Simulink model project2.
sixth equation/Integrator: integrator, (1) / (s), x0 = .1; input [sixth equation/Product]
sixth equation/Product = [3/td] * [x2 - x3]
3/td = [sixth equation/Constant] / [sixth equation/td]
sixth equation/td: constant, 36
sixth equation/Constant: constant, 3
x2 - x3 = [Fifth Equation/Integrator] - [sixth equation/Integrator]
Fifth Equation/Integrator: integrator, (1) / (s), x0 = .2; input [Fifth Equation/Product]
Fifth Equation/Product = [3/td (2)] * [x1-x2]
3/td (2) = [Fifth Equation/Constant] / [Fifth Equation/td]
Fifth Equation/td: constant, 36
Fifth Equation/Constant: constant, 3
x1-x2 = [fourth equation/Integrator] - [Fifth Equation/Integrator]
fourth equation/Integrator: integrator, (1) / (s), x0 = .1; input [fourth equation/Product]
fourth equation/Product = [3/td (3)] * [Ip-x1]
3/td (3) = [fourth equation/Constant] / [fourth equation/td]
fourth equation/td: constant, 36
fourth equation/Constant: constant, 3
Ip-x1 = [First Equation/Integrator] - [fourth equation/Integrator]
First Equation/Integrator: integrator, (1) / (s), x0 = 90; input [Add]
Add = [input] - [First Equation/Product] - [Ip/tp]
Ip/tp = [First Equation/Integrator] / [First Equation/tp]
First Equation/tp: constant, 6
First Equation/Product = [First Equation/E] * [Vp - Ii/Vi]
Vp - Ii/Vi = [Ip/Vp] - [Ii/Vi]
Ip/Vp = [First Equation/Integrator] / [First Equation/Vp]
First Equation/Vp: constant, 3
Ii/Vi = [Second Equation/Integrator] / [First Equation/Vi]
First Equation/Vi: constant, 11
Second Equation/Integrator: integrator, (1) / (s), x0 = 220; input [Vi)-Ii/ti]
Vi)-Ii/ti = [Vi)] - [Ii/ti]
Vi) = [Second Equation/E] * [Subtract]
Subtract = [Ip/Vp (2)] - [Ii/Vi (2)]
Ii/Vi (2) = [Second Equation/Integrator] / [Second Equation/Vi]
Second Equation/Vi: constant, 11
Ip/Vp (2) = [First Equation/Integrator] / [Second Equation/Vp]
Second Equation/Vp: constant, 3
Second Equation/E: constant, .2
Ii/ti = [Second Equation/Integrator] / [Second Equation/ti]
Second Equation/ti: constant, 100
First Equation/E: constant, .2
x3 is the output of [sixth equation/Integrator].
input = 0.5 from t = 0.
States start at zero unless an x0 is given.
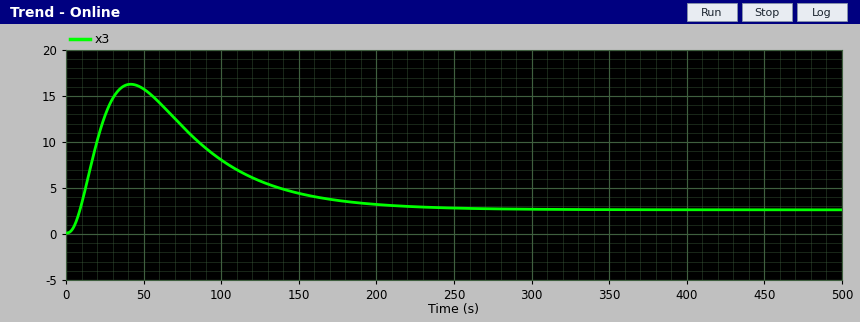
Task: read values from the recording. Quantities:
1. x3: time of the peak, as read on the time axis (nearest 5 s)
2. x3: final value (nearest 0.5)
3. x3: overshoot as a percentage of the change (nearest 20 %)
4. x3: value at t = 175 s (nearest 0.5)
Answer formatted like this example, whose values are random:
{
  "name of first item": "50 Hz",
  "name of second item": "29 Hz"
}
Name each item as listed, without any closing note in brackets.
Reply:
{
  "x3: time of the peak, as read on the time axis": "40 s",
  "x3: final value": "2.5",
  "x3: overshoot as a percentage of the change": "540 %",
  "x3: value at t = 175 s": "3.5"
}
